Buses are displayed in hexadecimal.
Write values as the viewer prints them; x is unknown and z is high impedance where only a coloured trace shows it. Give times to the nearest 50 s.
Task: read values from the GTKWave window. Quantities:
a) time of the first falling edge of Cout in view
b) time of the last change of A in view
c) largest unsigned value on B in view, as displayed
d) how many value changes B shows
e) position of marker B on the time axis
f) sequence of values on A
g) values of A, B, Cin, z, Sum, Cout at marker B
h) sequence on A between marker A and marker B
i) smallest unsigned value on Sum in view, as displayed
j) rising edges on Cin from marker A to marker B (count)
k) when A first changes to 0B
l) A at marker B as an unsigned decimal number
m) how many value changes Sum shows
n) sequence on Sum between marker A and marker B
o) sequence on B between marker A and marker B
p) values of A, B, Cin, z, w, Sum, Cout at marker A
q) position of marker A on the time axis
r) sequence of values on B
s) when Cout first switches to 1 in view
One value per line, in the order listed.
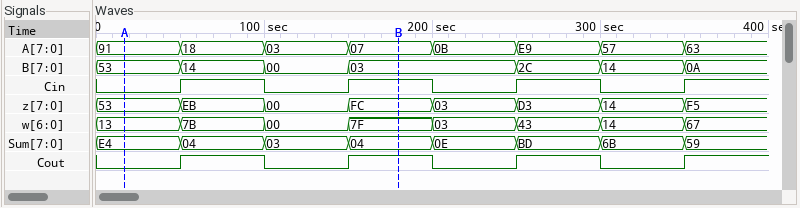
100 s
350 s
53
6
200 s
91, 18, 03, 07, 0B, E9, 57, 63
A=07, B=03, Cin=1, z=FC, Sum=04, Cout=1
91, 18, 03, 07
03
2
200 s
7
7
E4, 04, 03, 04
53, 14, 00, 03
A=91, B=53, Cin=0, z=53, w=13, Sum=E4, Cout=0
0 s
53, 14, 00, 03, 2C, 14, 0A
50 s
